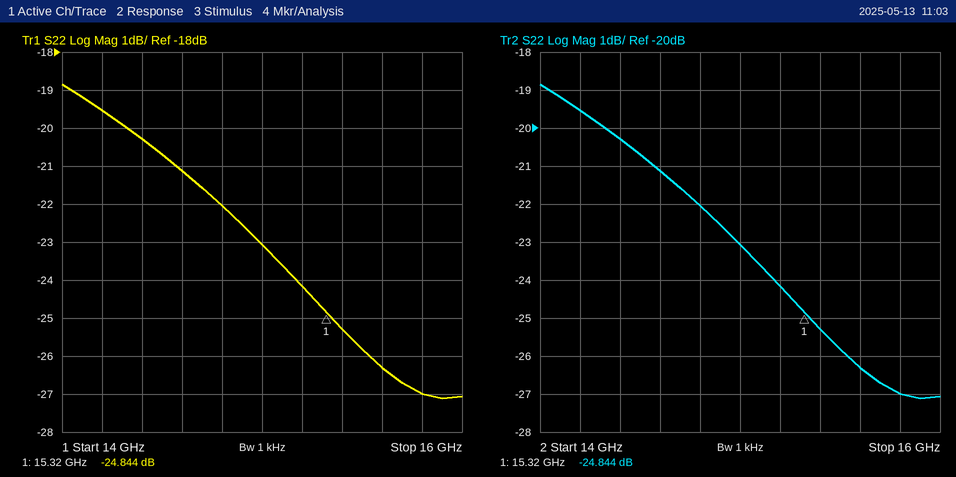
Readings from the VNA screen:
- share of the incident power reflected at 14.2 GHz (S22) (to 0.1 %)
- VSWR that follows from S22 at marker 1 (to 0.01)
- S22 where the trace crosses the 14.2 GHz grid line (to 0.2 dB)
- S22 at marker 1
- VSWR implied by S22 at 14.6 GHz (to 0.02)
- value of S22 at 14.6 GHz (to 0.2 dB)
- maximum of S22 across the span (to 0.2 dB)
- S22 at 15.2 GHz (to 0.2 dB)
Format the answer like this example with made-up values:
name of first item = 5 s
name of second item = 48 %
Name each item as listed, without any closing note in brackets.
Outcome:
share of the incident power reflected at 14.2 GHz (S22) = 1.1 %
VSWR that follows from S22 at marker 1 = 1.12
S22 where the trace crosses the 14.2 GHz grid line = -19.6 dB
S22 at marker 1 = -24.844 dB
VSWR implied by S22 at 14.6 GHz = 1.20
value of S22 at 14.6 GHz = -21.2 dB
maximum of S22 across the span = -18.8 dB
S22 at 15.2 GHz = -24.2 dB
